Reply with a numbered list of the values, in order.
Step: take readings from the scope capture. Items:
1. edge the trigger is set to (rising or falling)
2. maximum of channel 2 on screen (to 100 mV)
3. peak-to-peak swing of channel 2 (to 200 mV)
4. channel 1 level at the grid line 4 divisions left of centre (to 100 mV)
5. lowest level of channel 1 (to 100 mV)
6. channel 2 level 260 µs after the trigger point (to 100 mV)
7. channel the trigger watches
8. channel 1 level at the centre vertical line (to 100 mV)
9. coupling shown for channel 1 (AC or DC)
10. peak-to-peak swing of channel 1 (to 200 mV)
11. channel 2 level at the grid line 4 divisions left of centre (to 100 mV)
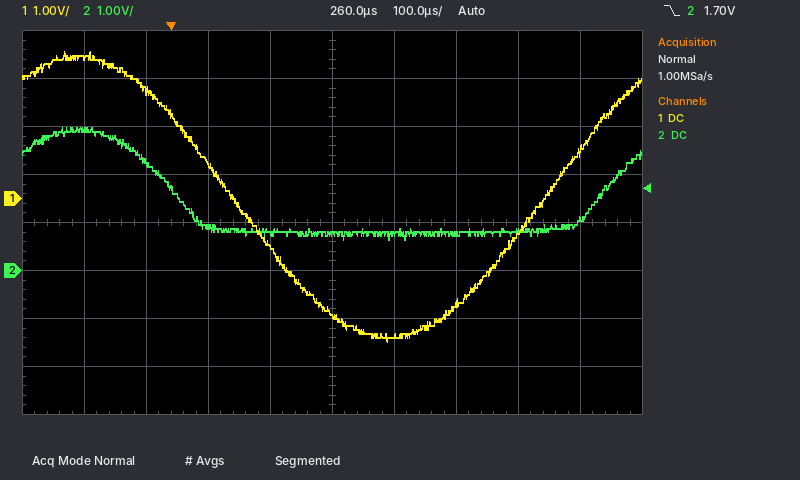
1. falling
2. 3.0 V
3. 2.4 V
4. 2.9 V
5. -3.0 V
6. 800 mV
7. channel 2
8. -2.4 V
9. DC
10. 6.0 V
11. 2.9 V
